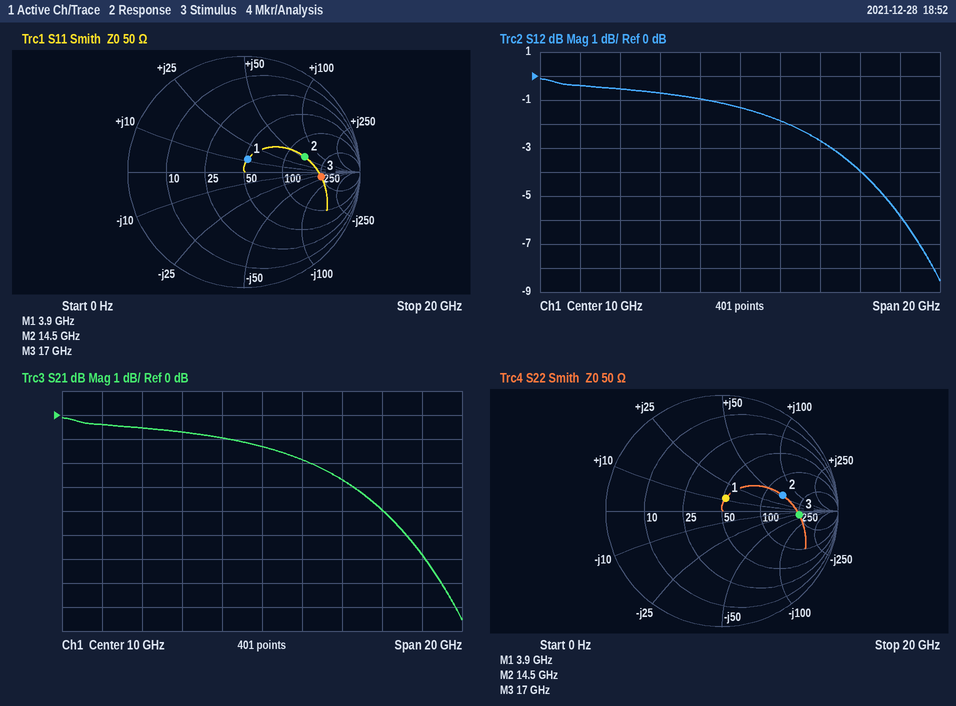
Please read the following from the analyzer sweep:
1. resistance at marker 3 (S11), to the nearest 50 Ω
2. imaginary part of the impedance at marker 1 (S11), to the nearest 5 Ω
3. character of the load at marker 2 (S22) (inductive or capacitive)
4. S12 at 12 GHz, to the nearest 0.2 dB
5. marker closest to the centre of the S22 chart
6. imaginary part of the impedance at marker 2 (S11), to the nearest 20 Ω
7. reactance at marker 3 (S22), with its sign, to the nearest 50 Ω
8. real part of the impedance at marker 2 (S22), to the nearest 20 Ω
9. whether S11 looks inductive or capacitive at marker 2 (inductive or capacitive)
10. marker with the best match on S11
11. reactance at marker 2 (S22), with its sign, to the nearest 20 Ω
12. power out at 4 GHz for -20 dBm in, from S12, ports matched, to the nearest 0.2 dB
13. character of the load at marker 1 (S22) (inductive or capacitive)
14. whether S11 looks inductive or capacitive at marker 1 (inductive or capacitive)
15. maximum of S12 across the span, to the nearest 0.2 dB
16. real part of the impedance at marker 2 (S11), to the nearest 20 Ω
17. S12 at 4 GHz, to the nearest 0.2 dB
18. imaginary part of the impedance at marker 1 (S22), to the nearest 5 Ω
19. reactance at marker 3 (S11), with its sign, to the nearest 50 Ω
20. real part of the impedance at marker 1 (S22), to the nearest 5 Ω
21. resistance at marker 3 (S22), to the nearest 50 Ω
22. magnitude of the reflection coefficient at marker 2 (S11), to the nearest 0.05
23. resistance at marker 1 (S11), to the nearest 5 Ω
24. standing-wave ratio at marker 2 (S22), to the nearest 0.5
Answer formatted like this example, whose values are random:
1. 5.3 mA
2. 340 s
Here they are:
1. 250 Ω
2. +10 Ω
3. inductive
4. -1.8 dB
5. marker 1
6. +60 Ω
7. -50 Ω
8. 140 Ω
9. inductive
10. marker 1
11. +60 Ω
12. -20.6 dBm
13. inductive
14. inductive
15. -0.2 dB
16. 140 Ω
17. -0.6 dB
18. +10 Ω
19. -50 Ω
20. 50 Ω
21. 250 Ω
22. 0.55
23. 50 Ω
24. 3.5
